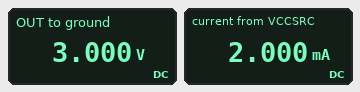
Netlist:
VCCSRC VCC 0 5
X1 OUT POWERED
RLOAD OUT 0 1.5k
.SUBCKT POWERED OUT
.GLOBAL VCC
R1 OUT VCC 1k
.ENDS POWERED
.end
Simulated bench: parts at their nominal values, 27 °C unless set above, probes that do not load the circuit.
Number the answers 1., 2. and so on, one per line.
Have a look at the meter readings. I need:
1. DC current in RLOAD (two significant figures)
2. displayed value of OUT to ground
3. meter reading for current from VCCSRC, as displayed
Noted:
1. 2.0 mA
2. 3.000 V
3. 2.000 mA
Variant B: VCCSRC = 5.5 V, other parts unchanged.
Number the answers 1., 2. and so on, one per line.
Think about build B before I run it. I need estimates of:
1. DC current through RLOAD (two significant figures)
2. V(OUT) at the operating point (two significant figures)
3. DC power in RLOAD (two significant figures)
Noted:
1. 2.2 mA
2. 3.3 V
3. 7.3 mW
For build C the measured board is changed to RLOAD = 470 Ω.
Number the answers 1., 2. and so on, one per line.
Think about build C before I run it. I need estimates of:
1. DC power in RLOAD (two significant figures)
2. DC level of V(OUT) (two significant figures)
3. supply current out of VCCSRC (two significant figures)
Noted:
1. 5.4 mW
2. 1.6 V
3. 3.4 mA
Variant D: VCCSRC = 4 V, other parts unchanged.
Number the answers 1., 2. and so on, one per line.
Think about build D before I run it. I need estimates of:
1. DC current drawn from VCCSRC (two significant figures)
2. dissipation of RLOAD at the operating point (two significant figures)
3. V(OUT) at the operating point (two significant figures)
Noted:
1. 1.6 mA
2. 3.8 mW
3. 2.4 V
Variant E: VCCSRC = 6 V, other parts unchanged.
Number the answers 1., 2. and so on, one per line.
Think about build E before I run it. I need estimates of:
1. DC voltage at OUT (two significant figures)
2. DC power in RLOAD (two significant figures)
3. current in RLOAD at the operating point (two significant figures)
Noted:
1. 3.6 V
2. 8.6 mW
3. 2.4 mA
